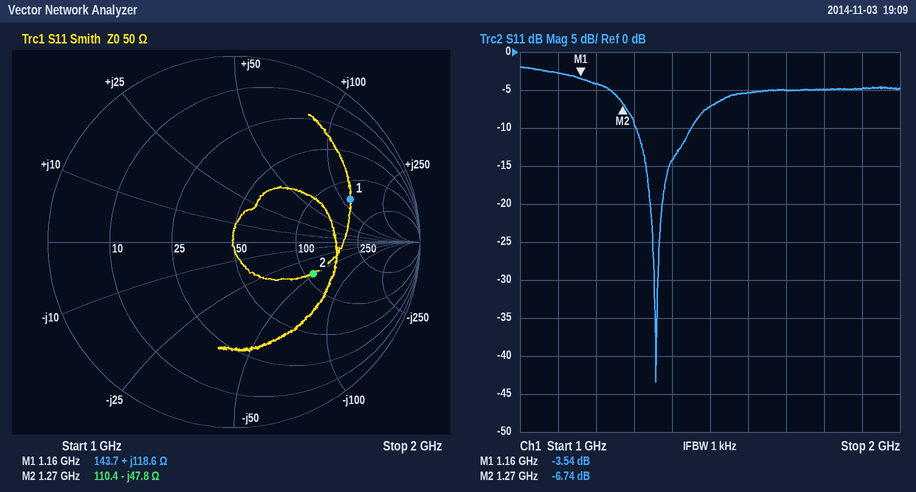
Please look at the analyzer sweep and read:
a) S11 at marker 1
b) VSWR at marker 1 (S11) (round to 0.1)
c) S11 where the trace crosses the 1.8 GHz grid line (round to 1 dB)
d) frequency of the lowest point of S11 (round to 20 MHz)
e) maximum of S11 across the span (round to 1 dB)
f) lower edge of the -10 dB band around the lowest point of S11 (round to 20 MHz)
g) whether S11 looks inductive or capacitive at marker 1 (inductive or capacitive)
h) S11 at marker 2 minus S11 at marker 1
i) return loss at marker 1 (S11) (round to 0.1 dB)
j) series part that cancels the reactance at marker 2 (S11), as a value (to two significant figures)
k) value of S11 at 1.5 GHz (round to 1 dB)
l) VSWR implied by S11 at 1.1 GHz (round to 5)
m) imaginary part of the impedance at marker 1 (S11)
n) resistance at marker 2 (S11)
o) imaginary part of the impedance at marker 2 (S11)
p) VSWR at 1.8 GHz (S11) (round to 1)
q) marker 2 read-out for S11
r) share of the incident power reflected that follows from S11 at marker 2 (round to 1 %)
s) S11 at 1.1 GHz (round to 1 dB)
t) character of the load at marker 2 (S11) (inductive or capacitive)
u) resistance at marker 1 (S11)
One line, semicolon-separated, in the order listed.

-3.54 dB; 5.0; -5 dB; 1.36 GHz; -2 dB; 1.30 GHz; inductive; -3.20 dB; 3.5 dB; 6.0 nH; -7 dB; 5; +118.6 Ω; 110.4 Ω; -47.8 Ω; 4; -6.74 dB; 21 %; -3 dB; capacitive; 143.7 Ω
